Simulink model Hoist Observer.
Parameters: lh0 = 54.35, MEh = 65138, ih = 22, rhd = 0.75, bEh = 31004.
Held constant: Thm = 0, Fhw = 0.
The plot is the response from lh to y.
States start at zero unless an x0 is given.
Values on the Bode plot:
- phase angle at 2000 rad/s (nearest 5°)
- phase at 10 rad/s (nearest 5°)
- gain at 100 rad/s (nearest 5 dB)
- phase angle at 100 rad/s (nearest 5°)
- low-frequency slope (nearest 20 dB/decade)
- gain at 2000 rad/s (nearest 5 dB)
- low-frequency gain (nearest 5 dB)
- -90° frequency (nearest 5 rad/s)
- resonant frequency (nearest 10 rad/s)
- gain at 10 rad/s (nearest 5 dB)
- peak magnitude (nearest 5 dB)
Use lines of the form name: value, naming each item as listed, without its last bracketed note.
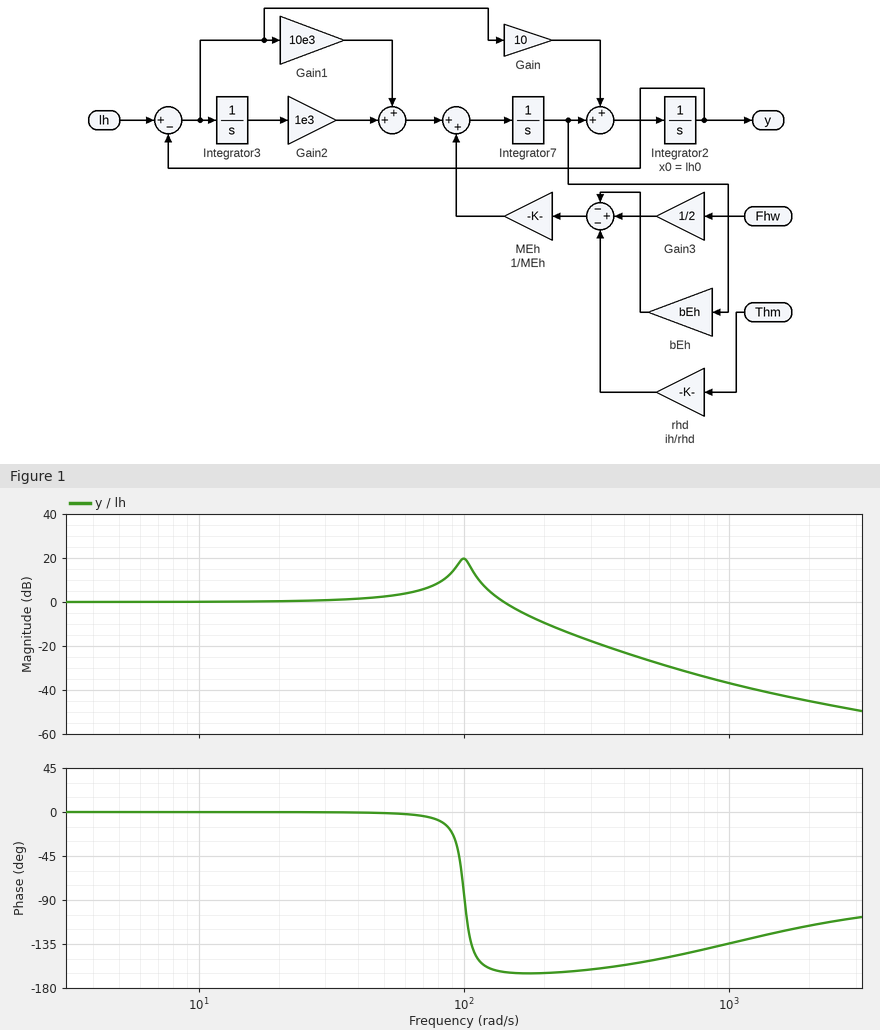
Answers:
phase angle at 2000 rad/s: -115°
phase at 10 rad/s: 0°
gain at 100 rad/s: 20 dB
phase angle at 100 rad/s: -85°
low-frequency slope: 0 dB/decade
gain at 2000 rad/s: -45 dB
low-frequency gain: 0 dB
-90° frequency: 100 rad/s
resonant frequency: 100 rad/s
gain at 10 rad/s: 0 dB
peak magnitude: 20 dB
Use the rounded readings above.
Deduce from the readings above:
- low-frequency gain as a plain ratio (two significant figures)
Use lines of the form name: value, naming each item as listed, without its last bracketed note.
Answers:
low-frequency gain as a plain ratio: 1.0
